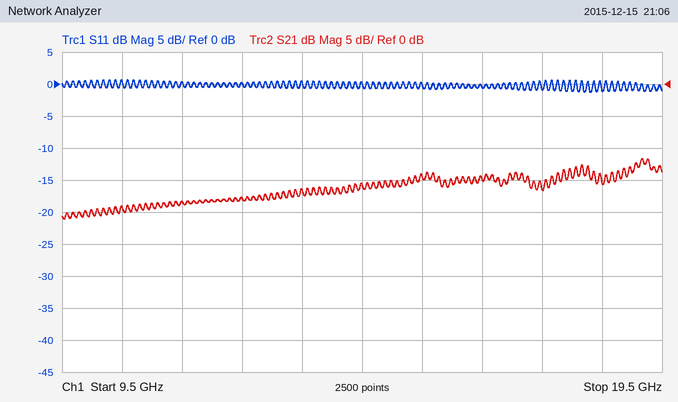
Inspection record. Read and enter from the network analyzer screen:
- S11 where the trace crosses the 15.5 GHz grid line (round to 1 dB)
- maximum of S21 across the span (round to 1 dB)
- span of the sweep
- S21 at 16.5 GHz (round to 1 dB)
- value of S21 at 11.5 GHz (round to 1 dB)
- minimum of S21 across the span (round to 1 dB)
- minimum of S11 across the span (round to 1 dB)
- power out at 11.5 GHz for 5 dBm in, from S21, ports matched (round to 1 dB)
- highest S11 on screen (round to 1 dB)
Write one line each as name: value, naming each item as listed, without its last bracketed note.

S11 where the trace crosses the 15.5 GHz grid line: 0 dB
maximum of S21 across the span: -12 dB
span of the sweep: 10 GHz
S21 at 16.5 GHz: -15 dB
value of S21 at 11.5 GHz: -18 dB
minimum of S21 across the span: -21 dB
minimum of S11 across the span: -1 dB
power out at 11.5 GHz for 5 dBm in, from S21, ports matched: -13 dBm
highest S11 on screen: 1 dB
